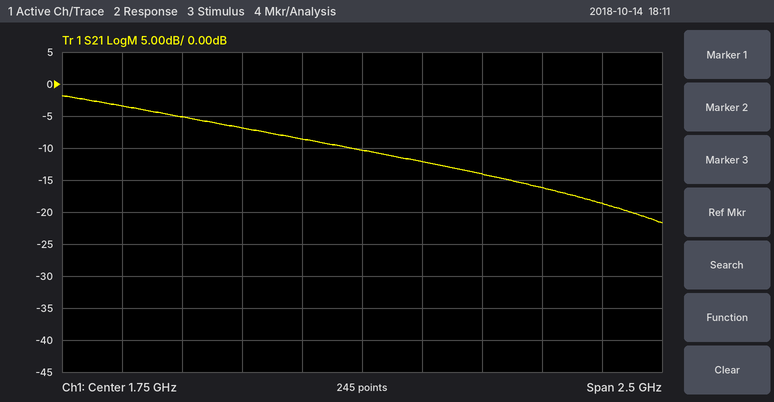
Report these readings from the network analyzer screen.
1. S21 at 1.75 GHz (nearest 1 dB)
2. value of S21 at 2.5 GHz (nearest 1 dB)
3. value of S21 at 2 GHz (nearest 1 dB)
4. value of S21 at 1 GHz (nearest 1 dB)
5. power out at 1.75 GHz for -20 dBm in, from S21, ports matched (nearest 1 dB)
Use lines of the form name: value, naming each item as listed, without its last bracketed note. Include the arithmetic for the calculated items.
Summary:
S21 at 1.75 GHz: -10 dB
value of S21 at 2.5 GHz: -16 dB
value of S21 at 2 GHz: -12 dB
value of S21 at 1 GHz: -5 dB
power out at 1.75 GHz for -20 dBm in, from S21, ports matched: -20 dBm + (-10 dB) = -30 dBm
